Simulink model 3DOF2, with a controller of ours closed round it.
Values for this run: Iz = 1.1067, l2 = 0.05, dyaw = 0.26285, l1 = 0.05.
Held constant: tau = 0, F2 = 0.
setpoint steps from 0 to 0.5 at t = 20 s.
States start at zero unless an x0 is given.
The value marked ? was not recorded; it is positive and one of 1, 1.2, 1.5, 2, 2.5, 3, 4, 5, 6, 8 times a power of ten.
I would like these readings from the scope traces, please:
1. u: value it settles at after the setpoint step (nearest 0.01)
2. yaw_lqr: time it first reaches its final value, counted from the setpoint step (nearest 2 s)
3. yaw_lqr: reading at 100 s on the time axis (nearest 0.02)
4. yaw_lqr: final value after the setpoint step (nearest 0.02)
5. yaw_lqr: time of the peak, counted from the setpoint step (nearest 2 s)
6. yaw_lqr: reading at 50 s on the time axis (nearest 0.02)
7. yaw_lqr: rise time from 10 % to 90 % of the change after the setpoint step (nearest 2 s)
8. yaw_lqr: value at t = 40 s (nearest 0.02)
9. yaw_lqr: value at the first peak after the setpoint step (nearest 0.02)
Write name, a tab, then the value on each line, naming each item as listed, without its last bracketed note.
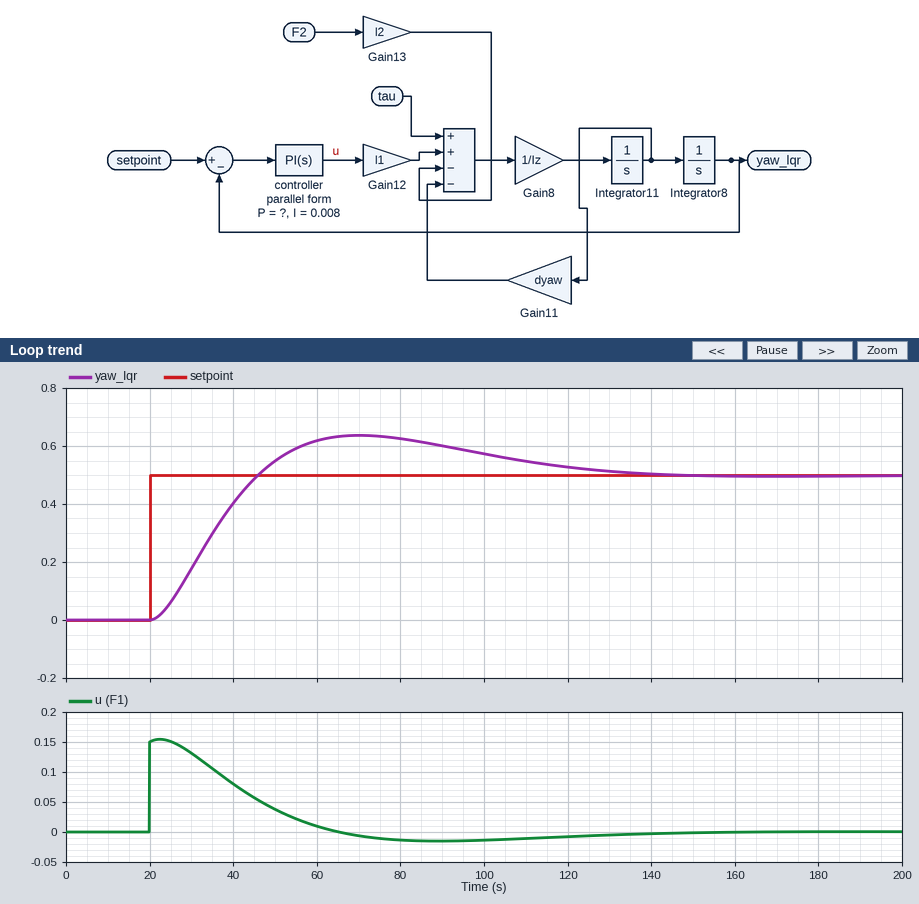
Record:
u: value it settles at after the setpoint step	0.00
yaw_lqr: time it first reaches its final value, counted from the setpoint step	26 s
yaw_lqr: reading at 100 s on the time axis	0.58
yaw_lqr: final value after the setpoint step	0.50
yaw_lqr: time of the peak, counted from the setpoint step	50 s
yaw_lqr: reading at 50 s on the time axis	0.54
yaw_lqr: rise time from 10 % to 90 % of the change after the setpoint step	18 s
yaw_lqr: value at t = 40 s	0.40
yaw_lqr: value at the first peak after the setpoint step	0.64
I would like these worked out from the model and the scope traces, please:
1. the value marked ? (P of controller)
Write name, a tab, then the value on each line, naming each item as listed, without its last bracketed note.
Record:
the value marked ?	0.3
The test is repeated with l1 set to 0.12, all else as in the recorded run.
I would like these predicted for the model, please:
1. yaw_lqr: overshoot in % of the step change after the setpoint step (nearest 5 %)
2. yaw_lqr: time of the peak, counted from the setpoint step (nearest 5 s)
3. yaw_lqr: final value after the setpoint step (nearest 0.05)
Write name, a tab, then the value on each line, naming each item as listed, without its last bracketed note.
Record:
yaw_lqr: overshoot in % of the step change after the setpoint step	25 %
yaw_lqr: time of the peak, counted from the setpoint step	25 s
yaw_lqr: final value after the setpoint step	0.50
